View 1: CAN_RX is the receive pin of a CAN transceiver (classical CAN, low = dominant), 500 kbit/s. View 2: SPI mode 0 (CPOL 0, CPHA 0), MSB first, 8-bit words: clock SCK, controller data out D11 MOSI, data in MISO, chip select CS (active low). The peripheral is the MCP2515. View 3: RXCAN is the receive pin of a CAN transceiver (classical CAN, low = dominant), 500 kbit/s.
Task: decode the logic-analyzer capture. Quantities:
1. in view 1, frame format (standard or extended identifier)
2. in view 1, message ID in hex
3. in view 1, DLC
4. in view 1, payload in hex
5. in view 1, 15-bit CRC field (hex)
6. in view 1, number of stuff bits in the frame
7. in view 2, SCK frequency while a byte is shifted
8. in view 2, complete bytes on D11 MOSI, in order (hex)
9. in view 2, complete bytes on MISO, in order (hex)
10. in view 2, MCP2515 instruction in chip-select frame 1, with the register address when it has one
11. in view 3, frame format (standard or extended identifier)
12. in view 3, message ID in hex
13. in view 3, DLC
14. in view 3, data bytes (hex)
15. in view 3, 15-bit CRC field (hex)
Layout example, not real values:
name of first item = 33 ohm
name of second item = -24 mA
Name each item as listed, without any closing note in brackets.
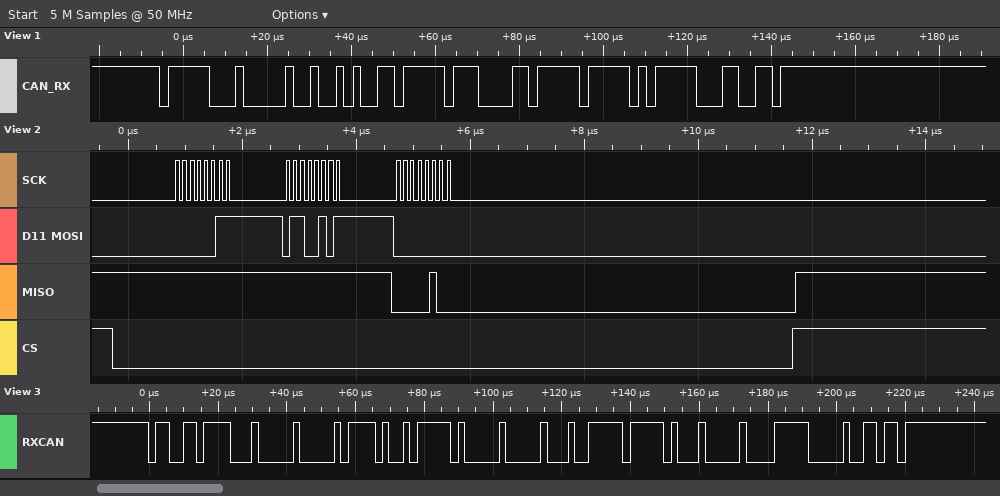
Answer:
in view 1, frame format = standard
in view 1, message ID in hex = 0x7C8
in view 1, DLC = 4
in view 1, payload in hex = A6 FF 0D FF
in view 1, 15-bit CRC field = 0x6F99
in view 1, number of stuff bits in the frame = 6
in view 2, SCK frequency while a byte is shifted = 8 MHz
in view 2, complete bytes on D11 MOSI, in order = 03 65 00
in view 2, complete bytes on MISO, in order = FF FF 04
in view 2, MCP2515 instruction in chip-select frame 1, with the register address when it has one = READ 0x65
in view 3, frame format = standard
in view 3, message ID in hex = 0x66F
in view 3, DLC = 8
in view 3, data bytes = 00 F4 BF 00 04 FF E2 00
in view 3, 15-bit CRC field = 0x7C0D
